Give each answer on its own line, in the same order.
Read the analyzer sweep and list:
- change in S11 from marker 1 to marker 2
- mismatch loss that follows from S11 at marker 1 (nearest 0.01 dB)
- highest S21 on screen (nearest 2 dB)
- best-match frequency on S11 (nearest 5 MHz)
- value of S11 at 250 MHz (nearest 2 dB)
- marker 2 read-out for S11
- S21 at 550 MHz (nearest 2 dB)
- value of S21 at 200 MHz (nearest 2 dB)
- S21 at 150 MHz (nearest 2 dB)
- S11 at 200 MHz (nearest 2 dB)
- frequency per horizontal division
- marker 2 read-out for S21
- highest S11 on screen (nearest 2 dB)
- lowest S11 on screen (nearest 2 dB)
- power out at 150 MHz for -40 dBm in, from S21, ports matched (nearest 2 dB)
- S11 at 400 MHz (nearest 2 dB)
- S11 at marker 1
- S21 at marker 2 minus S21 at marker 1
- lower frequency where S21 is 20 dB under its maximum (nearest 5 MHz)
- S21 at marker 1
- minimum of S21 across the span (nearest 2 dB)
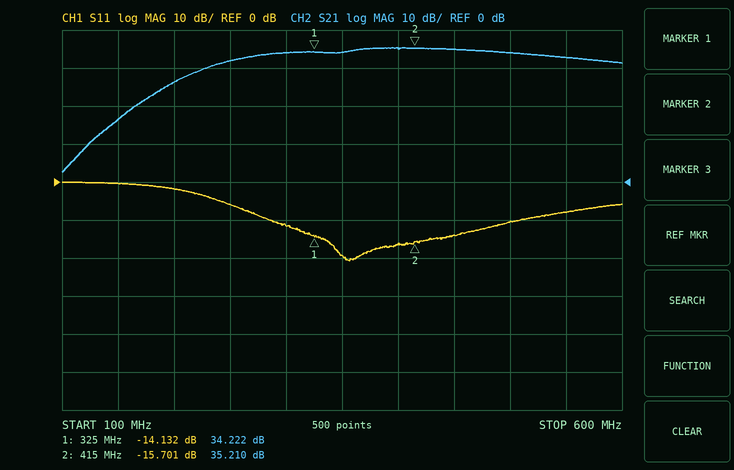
-1.569 dB
0.17 dB
36 dB
355 MHz
-6 dB
-15.701 dB
32 dB
26 dB
16 dB
-2 dB
50 MHz
35.210 dB
0 dB
-20 dB
-24 dBm
-16 dB
-14.132 dB
0.988 dB
145 MHz
34.222 dB
2 dB
